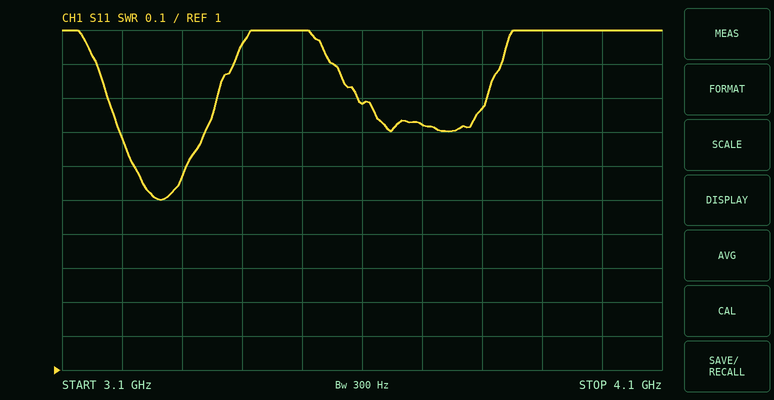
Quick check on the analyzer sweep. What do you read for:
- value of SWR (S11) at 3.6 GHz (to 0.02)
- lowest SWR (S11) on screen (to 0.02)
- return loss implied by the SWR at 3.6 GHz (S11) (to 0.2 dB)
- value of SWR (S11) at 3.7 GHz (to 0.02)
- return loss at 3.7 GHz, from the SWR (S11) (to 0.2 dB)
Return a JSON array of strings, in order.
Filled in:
["1.78", "1.50", "11.0 dB", "1.72", "11.6 dB"]
